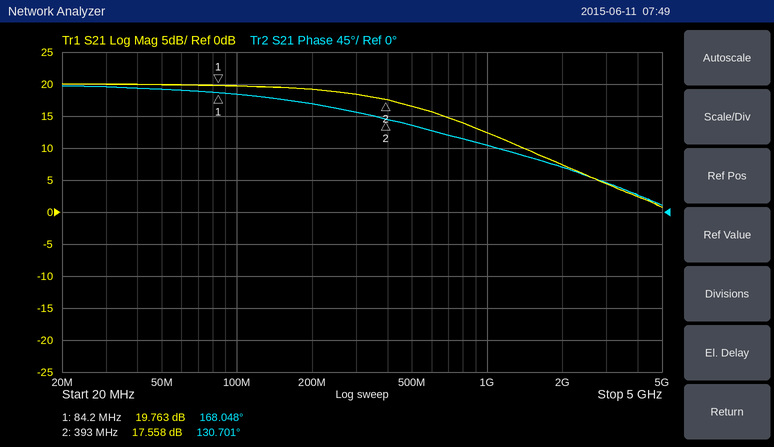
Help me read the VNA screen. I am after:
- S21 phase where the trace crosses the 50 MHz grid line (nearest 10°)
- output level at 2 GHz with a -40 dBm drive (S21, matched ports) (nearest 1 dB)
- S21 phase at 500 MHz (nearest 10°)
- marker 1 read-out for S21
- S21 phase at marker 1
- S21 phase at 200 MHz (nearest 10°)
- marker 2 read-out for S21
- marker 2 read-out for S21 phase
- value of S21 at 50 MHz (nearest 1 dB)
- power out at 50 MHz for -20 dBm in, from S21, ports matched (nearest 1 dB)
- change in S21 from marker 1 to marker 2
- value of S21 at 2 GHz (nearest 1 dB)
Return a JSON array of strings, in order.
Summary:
["170°", "-33 dBm", "120°", "19.763 dB", "168.048°", "150°", "17.558 dB", "130.701°", "20 dB", "0 dBm", "-2.205 dB", "7 dB"]
